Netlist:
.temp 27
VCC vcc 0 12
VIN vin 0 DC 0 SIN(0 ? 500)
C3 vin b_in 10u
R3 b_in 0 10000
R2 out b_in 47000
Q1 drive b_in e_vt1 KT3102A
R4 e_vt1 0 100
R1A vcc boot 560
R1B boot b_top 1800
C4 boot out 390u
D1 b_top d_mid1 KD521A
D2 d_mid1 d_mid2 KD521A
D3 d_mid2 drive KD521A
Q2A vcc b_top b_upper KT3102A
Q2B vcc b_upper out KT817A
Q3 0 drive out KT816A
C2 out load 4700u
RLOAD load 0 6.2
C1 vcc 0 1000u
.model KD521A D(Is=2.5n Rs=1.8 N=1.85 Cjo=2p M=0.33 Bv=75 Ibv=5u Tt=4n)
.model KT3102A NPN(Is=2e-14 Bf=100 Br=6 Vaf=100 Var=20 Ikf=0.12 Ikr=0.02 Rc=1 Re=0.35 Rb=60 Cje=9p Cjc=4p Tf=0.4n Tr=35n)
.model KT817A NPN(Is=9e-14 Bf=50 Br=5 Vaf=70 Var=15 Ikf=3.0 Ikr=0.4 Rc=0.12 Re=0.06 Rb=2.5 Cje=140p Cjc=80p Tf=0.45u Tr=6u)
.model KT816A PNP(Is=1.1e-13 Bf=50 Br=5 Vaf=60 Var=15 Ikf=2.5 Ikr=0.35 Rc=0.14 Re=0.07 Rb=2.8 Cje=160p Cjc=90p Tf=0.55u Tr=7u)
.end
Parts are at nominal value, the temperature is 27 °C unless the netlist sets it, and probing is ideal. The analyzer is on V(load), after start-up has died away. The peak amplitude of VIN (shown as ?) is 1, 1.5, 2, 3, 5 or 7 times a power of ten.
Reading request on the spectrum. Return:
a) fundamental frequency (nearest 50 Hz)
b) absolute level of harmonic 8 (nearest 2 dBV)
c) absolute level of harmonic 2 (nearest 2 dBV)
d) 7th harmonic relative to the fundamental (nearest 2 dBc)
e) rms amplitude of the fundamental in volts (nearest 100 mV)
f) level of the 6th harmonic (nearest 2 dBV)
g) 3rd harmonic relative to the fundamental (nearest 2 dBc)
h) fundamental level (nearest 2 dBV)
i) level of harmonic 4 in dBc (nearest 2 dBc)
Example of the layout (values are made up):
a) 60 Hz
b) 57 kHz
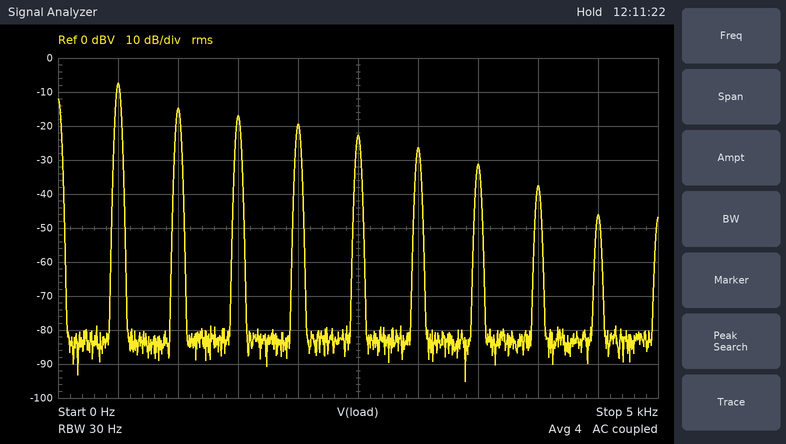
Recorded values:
a) 500 Hz
b) -38 dBV
c) -14 dBV
d) -24 dBc
e) 400 mV
f) -26 dBV
g) -10 dBc
h) -8 dBV
i) -12 dBc
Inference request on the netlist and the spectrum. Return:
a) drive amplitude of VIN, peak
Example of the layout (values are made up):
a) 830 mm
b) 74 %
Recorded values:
a) 100 mV
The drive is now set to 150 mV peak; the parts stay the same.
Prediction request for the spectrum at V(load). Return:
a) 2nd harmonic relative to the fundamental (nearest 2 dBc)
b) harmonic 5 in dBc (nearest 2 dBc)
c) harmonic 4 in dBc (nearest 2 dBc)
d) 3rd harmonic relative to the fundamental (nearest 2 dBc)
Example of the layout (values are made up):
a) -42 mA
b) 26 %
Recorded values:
a) -6 dBc
b) -14 dBc
c) -10 dBc
d) -8 dBc
